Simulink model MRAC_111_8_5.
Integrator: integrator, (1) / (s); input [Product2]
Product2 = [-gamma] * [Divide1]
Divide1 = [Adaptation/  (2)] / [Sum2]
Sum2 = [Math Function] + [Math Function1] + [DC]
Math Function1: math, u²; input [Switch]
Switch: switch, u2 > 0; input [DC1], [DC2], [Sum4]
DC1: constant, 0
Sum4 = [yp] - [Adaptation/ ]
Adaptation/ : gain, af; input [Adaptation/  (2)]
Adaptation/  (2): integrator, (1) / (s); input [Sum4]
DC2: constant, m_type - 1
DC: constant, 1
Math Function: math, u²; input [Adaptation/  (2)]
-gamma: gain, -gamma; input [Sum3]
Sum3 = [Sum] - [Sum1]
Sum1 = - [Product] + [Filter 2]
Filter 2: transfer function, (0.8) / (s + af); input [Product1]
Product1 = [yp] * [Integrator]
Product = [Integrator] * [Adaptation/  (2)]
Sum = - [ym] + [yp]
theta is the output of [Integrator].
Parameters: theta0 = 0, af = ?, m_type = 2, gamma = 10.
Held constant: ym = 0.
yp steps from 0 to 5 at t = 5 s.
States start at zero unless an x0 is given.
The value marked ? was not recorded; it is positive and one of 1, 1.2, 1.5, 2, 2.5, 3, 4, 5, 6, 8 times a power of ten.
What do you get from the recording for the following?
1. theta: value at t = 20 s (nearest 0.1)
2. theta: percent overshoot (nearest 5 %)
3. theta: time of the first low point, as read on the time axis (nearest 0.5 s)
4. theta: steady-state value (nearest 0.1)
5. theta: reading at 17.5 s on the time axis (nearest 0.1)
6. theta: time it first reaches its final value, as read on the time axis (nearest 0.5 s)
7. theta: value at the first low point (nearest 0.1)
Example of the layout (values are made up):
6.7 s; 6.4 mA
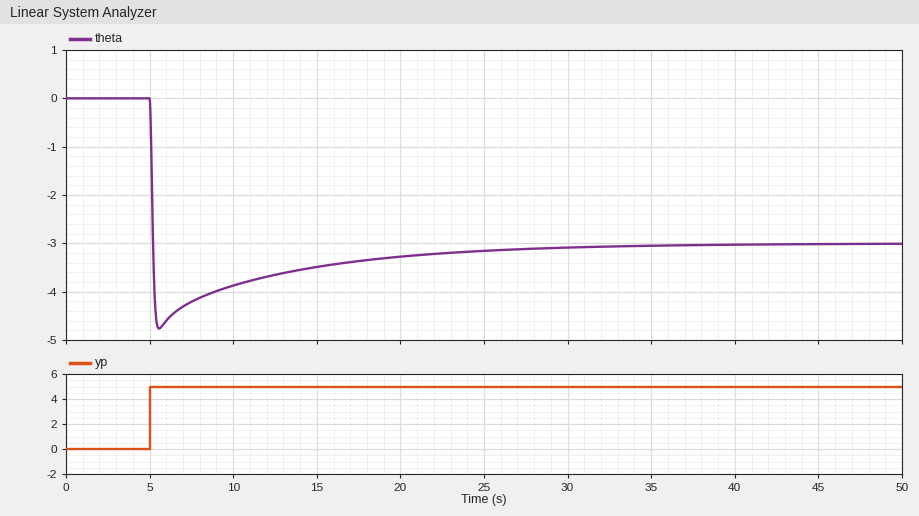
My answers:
-3.3; 60 %; 5.5 s; -3.0; -3.4; 5.0 s; -4.8
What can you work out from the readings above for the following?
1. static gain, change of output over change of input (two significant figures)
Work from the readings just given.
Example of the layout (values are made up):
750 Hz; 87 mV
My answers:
-0.60
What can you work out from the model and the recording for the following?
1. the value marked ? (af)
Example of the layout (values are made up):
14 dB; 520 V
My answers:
0.6
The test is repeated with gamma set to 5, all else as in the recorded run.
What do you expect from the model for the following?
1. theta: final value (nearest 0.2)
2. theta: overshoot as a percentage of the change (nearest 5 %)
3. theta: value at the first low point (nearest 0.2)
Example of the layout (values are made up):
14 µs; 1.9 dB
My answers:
-3.0; 20 %; -3.6
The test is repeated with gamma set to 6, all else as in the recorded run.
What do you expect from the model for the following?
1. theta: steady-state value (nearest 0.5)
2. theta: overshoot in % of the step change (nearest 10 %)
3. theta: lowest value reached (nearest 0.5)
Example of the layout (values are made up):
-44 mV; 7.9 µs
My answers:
-3.0; 30 %; -4.0
